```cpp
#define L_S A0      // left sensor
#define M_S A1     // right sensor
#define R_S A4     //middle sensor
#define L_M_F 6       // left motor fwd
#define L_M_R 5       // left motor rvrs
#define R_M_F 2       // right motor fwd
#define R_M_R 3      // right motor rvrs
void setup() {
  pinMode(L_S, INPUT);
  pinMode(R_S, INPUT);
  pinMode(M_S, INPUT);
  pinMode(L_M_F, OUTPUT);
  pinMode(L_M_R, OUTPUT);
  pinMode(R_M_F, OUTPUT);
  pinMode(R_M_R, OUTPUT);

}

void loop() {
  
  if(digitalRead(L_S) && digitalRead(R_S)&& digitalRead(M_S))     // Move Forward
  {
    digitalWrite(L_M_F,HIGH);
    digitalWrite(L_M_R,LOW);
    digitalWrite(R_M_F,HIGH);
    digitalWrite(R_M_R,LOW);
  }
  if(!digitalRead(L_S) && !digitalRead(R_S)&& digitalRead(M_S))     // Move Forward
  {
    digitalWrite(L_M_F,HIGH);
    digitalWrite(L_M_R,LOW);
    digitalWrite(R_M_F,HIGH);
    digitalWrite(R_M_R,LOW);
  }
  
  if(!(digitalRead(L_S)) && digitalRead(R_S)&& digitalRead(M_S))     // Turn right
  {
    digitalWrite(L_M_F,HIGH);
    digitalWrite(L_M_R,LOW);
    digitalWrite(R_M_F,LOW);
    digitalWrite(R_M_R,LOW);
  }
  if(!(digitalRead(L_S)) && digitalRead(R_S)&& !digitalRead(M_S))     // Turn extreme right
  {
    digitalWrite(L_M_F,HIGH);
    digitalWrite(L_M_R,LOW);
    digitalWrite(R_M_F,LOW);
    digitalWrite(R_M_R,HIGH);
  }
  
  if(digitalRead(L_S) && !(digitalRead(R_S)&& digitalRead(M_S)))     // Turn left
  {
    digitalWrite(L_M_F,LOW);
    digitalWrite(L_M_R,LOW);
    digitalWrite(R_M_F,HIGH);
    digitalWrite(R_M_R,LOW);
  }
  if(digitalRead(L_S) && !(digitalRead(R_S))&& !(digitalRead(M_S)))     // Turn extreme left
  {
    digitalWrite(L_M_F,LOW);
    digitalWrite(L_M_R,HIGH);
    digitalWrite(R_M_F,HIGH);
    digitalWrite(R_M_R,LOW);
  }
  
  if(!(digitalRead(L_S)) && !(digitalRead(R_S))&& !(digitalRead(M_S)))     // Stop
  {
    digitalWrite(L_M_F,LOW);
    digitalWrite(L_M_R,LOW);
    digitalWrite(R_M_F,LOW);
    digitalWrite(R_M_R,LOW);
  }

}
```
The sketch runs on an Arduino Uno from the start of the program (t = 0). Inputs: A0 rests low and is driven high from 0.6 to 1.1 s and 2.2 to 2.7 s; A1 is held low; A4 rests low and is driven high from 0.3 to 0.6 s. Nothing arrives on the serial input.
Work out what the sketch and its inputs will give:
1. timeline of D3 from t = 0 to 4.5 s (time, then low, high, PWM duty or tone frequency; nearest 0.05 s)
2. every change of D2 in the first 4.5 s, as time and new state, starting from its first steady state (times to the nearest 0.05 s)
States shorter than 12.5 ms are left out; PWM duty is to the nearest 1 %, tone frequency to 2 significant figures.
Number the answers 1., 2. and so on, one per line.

1. 0 s low; 0.3 s high; 0.6 s low
2. 0 s low; 0.6 s high; 1.1 s low; 2.2 s high; 2.7 s low
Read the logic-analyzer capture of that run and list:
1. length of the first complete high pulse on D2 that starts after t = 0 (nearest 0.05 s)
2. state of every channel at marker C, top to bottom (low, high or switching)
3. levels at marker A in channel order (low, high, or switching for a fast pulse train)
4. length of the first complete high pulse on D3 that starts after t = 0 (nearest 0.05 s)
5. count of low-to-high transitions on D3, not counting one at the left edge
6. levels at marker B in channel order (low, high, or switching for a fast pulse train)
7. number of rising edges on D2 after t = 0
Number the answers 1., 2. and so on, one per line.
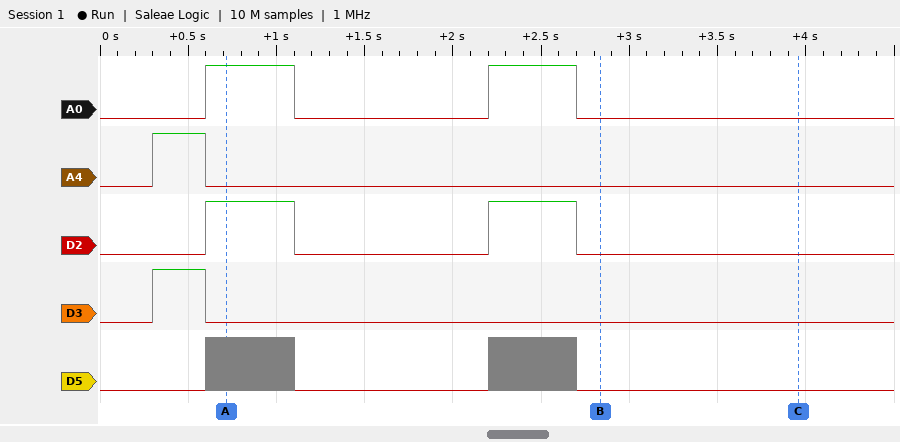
1. 0.50 s
2. A0 low, A4 low, D2 low, D3 low, D5 low
3. A0 high, A4 low, D2 high, D3 low, D5 switching
4. 0.30 s
5. 1
6. A0 low, A4 low, D2 low, D3 low, D5 low
7. 2
